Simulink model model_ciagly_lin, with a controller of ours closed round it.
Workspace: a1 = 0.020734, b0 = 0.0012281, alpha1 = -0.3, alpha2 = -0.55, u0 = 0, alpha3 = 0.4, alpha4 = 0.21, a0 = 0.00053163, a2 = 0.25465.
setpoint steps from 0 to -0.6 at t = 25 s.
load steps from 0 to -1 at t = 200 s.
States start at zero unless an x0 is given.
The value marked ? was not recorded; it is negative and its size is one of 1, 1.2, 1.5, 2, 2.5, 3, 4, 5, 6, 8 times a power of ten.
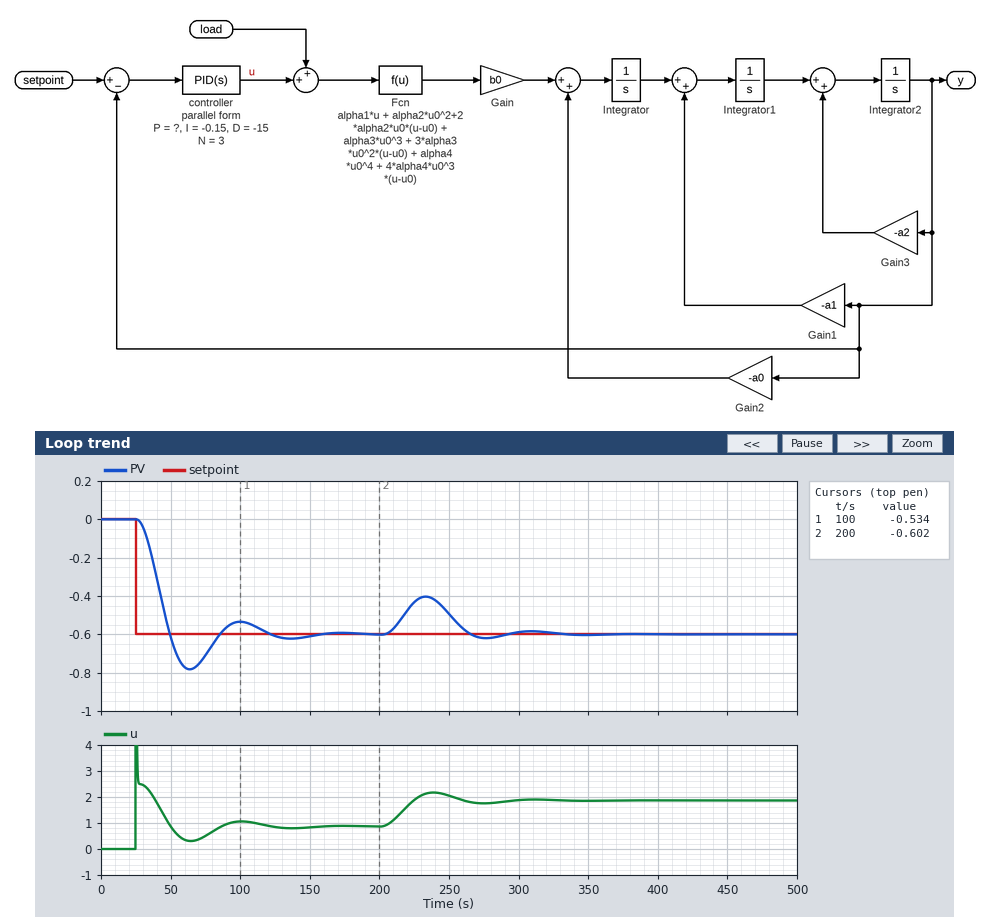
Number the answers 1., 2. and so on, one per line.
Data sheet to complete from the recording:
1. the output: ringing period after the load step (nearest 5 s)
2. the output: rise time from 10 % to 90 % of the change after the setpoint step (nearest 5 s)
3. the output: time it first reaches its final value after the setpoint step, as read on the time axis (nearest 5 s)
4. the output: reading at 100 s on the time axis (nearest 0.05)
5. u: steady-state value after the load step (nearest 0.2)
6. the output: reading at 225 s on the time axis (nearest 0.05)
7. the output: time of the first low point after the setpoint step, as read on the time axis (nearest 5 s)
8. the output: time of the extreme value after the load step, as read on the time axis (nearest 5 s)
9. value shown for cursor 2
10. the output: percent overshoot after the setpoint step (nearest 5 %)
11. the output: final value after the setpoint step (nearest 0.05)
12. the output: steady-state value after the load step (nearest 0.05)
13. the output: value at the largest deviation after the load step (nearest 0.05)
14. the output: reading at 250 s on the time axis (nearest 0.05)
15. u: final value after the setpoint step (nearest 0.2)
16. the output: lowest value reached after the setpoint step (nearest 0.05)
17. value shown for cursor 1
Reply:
1. 75 s
2. 15 s
3. 50 s
4. -0.55
5. 1.8
6. -0.45
7. 65 s
8. 235 s
9. -0.602
10. 30 %
11. -0.60
12. -0.60
13. -0.40
14. -0.50
15. 0.8
16. -0.80
17. -0.534
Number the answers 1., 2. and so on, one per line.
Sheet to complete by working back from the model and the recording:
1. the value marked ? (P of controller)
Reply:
1. -4
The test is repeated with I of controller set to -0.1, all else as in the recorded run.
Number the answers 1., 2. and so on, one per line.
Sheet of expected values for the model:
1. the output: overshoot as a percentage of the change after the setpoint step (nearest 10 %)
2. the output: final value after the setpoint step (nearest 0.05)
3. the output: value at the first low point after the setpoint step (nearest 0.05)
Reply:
1. 20 %
2. -0.60
3. -0.70
